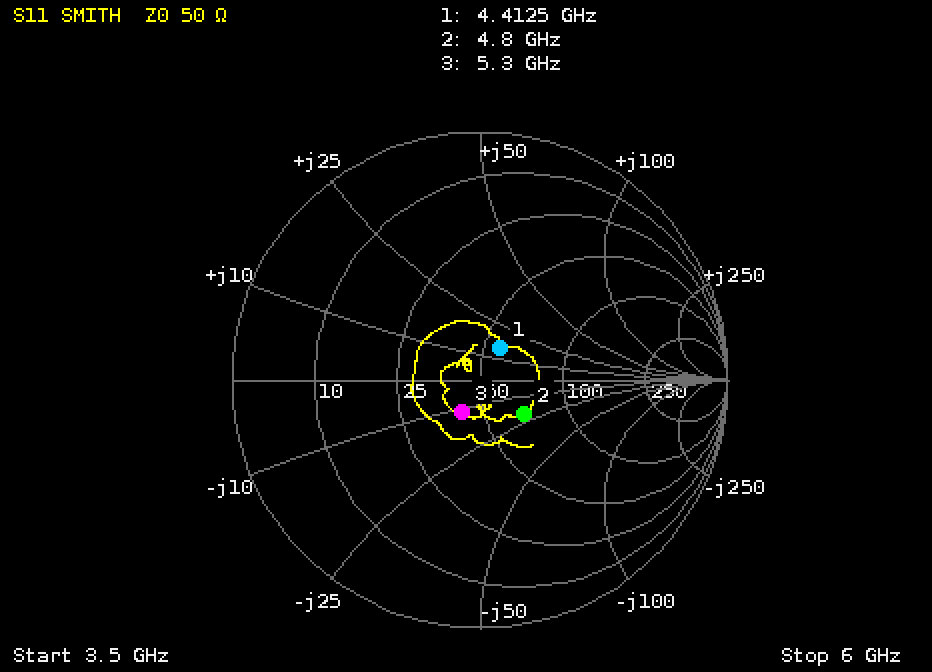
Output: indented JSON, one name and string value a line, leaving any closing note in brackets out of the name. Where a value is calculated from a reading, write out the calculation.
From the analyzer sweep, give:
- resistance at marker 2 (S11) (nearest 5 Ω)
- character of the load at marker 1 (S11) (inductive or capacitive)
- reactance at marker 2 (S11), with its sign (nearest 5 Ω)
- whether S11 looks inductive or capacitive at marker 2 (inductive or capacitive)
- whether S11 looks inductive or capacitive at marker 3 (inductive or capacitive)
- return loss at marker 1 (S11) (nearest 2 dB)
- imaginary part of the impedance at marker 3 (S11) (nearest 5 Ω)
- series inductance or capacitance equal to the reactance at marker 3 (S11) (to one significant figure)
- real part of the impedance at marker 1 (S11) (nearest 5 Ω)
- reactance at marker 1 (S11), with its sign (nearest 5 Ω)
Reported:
{
  "resistance at marker 2 (S11)": "70 Ω",
  "character of the load at marker 1 (S11)": "inductive",
  "reactance at marker 2 (S11), with its sign": "-20 Ω",
  "whether S11 looks inductive or capacitive at marker 2": "capacitive",
  "whether S11 looks inductive or capacitive at marker 3": "capacitive",
  "return loss at marker 1 (S11)": "16 dB",
  "imaginary part of the impedance at marker 3 (S11)": "-10 Ω",
  "series inductance or capacitance equal to the reactance at marker 3 (S11)": "C = 1/(2π × 5.3 GHz × 10 Ω) ≈ 3 pF",
  "real part of the impedance at marker 1 (S11)": "55 Ω",
  "reactance at marker 1 (S11), with its sign": "+15 Ω"
}
